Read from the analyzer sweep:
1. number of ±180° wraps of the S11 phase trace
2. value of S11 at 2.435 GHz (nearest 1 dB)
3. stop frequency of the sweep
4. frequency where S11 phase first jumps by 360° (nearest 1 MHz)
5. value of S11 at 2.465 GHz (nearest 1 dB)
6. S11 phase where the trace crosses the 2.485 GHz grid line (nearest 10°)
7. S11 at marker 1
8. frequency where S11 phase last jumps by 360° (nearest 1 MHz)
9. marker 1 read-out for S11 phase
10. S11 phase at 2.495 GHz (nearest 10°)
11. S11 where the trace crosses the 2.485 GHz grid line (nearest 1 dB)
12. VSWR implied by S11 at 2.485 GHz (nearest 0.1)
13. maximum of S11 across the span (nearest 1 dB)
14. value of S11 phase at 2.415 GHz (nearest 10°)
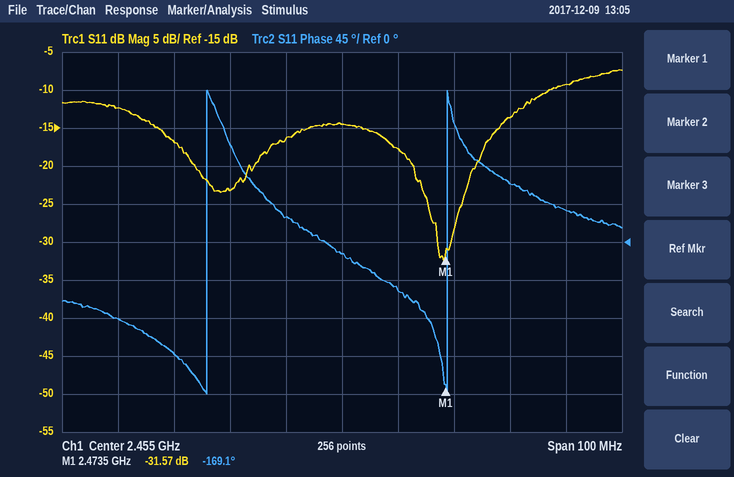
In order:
2
-23 dB
2.505 GHz
2.431 GHz
-18 dB
70°
-31.57 dB
2.474 GHz
-169.1°
40°
-14 dB
1.5
-7 dB
-90°
